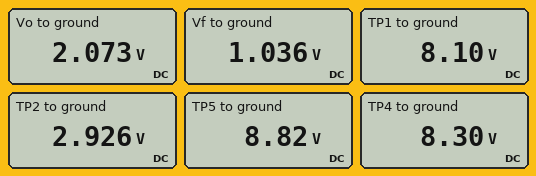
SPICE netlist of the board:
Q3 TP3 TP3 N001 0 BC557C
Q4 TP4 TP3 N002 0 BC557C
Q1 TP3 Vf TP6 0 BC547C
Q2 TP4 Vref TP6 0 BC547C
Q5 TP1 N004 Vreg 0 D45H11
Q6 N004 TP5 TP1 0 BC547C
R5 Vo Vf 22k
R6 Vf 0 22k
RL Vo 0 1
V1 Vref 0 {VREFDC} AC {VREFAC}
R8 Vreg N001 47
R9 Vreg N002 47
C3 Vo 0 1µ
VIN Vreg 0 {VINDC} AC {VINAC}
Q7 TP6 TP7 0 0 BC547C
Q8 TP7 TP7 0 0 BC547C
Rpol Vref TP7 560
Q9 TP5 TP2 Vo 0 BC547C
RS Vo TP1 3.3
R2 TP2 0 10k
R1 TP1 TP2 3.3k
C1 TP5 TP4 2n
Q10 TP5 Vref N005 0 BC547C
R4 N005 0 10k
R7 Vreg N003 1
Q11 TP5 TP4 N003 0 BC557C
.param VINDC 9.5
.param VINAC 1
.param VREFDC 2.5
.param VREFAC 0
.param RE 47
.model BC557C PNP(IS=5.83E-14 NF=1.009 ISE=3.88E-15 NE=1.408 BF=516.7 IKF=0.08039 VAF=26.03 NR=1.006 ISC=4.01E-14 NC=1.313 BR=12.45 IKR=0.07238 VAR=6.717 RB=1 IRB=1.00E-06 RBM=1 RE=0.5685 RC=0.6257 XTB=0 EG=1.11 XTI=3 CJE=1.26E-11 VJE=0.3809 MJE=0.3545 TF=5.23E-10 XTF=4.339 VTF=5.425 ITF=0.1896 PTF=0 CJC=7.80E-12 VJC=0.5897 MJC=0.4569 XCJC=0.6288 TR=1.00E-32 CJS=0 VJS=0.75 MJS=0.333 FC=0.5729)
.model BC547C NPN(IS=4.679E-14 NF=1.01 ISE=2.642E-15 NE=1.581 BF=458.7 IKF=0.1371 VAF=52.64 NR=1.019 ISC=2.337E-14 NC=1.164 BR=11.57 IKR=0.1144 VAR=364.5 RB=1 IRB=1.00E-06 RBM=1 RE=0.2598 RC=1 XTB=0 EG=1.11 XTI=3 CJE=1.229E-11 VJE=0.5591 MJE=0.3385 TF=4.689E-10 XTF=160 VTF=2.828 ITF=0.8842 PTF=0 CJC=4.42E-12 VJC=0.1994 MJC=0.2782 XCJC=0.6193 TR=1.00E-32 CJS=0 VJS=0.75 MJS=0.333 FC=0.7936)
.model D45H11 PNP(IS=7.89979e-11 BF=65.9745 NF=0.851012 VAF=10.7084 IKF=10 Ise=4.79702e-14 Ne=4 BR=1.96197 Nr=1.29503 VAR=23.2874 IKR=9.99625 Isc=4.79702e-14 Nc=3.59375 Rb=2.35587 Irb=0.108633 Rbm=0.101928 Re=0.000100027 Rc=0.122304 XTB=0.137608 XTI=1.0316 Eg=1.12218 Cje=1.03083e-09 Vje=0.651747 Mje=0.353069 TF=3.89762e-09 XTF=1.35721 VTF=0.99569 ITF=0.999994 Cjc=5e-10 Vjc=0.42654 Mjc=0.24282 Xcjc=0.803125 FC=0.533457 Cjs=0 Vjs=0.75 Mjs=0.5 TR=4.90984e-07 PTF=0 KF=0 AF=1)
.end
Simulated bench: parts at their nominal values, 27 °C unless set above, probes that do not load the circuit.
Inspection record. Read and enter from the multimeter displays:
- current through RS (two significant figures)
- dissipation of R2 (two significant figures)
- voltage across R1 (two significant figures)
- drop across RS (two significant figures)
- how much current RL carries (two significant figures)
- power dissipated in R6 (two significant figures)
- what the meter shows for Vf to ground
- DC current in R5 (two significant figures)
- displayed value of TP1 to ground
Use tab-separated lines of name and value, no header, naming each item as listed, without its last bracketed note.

current through RS	1.8 A
dissipation of R2	860 µW
voltage across R1	5.2 V
drop across RS	6.0 V
how much current RL carries	2.1 A
power dissipated in R6	49 µW
what the meter shows for Vf to ground	1.036 V
DC current in R5	47 µA
displayed value of TP1 to ground	8.10 V
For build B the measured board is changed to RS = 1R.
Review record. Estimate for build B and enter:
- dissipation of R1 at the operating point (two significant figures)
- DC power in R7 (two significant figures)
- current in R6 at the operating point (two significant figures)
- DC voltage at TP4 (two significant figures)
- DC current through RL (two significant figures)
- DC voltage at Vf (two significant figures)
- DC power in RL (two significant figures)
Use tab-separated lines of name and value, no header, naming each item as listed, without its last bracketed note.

dissipation of R1 at the operating point	3.3 mW
DC power in R7	18 mW
current in R6 at the operating point	96 µA
DC voltage at TP4	8.5 V
DC current through RL	4.2 A
DC voltage at Vf	2.1 V
DC power in RL	18 W
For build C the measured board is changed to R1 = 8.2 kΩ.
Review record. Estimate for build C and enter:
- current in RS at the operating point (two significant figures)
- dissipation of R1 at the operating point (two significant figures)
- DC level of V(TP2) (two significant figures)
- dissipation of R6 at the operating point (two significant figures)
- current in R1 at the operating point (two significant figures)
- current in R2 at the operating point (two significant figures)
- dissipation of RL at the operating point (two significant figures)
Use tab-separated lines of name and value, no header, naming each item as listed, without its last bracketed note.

current in RS at the operating point	1.9 A
dissipation of R1 at the operating point	3.8 mW
DC level of V(TP2)	2.8 V
dissipation of R6 at the operating point	48 µW
current in R1 at the operating point	680 µA
current in R2 at the operating point	280 µA
dissipation of RL at the operating point	4.2 W
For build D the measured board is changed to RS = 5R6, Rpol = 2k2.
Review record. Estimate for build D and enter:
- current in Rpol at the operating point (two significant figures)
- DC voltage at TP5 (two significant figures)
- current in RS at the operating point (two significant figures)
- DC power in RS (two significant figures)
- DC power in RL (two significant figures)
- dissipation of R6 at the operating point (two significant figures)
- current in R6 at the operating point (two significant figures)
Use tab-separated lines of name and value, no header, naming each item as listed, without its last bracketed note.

current in Rpol at the operating point	860 µA
DC voltage at TP5	5.0 V
current in RS at the operating point	630 mA
DC power in RS	2.2 W
DC power in RL	620 mW
dissipation of R6 at the operating point	7.0 µW
current in R6 at the operating point	18 µA
